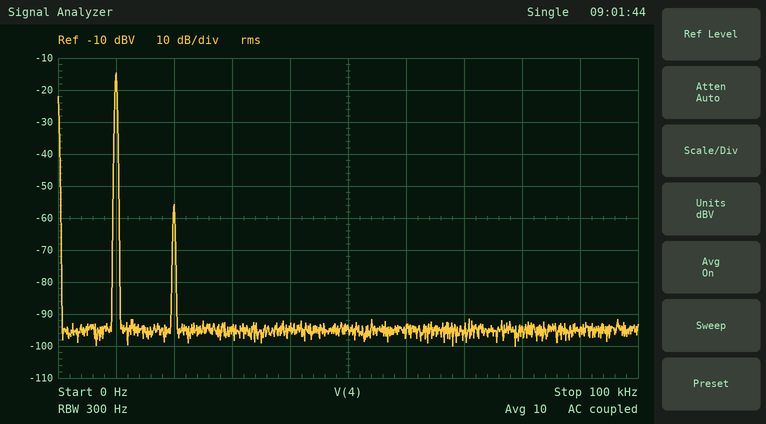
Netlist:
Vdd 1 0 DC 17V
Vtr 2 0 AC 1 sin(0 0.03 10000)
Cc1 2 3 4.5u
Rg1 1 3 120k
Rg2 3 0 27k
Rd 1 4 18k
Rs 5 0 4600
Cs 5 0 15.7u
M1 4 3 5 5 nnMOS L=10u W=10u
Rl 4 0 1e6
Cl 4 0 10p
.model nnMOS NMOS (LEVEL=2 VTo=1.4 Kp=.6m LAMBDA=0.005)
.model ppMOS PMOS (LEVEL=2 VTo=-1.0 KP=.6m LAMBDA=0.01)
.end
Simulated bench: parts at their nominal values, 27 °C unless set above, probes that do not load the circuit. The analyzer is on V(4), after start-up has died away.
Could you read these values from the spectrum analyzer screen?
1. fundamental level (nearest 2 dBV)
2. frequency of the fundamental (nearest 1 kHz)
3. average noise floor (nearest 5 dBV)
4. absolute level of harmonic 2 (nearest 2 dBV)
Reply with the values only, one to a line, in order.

-14 dBV
10 kHz
-95 dBV
-56 dBV
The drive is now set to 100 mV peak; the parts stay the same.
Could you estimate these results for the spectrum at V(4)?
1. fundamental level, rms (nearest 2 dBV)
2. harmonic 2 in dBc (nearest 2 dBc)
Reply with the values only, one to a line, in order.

-4 dBV
-30 dBc
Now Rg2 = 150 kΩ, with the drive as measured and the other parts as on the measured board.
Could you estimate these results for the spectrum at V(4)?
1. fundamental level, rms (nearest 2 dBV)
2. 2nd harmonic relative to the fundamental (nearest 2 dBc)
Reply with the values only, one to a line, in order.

-58 dBV
-50 dBc
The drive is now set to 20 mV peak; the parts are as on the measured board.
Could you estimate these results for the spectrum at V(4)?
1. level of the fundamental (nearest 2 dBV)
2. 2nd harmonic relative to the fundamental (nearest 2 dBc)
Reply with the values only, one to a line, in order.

-18 dBV
-44 dBc
